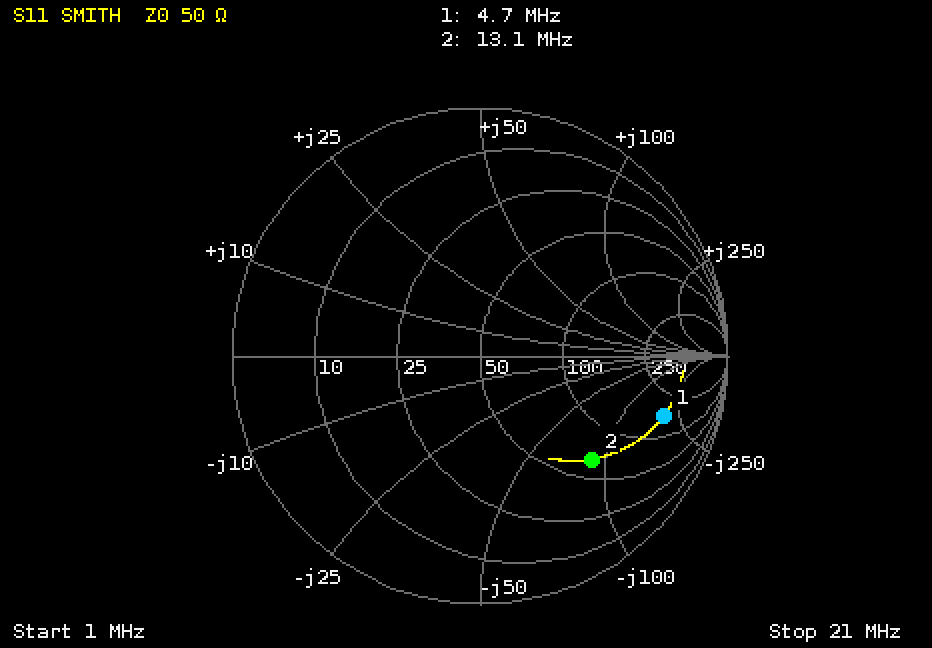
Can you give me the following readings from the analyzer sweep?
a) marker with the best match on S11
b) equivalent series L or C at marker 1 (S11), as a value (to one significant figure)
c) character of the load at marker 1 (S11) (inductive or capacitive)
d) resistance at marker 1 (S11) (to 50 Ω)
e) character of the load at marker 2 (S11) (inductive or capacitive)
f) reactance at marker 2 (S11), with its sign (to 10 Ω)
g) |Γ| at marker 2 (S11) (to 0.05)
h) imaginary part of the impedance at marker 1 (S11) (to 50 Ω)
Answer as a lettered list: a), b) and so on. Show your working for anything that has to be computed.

a) marker 2
b) C = 1/(2π × 4.7 MHz × 200 Ω) ≈ 169 pF, so 200 pF to one significant figure
c) capacitive
d) 150 Ω
e) capacitive
f) -90 Ω
g) 0.60
h) -200 Ω
